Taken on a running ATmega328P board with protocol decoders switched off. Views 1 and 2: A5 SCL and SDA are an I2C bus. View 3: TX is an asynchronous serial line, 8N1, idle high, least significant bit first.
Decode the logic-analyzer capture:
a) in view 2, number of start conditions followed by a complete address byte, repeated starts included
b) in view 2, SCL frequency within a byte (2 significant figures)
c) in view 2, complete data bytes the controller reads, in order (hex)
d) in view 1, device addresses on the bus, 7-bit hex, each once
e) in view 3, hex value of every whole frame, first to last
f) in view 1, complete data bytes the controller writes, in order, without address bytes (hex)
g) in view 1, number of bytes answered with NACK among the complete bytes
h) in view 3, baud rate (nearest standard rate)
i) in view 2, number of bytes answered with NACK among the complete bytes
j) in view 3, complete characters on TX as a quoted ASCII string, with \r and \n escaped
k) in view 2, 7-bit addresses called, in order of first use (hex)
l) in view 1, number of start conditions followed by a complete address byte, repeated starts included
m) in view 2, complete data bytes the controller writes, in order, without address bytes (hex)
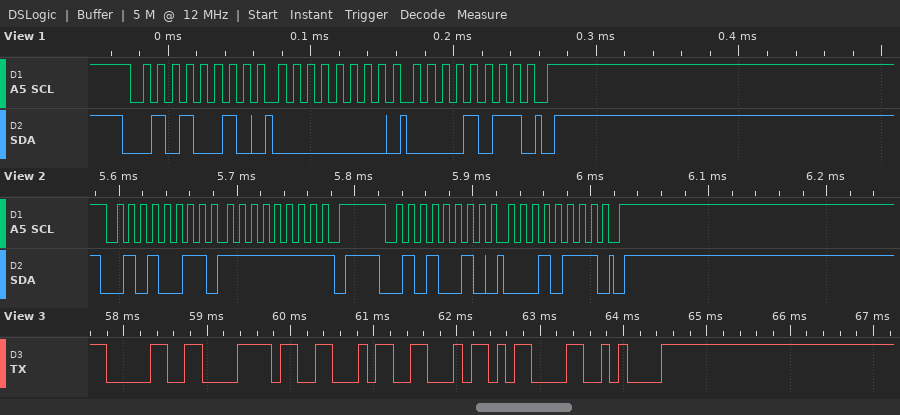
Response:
2
100 kHz
FF
0x29
30 78 46 46 0D 0A
00 0B
0
9600 baud
1
"0xFF\r\n"
0x29
1
17
